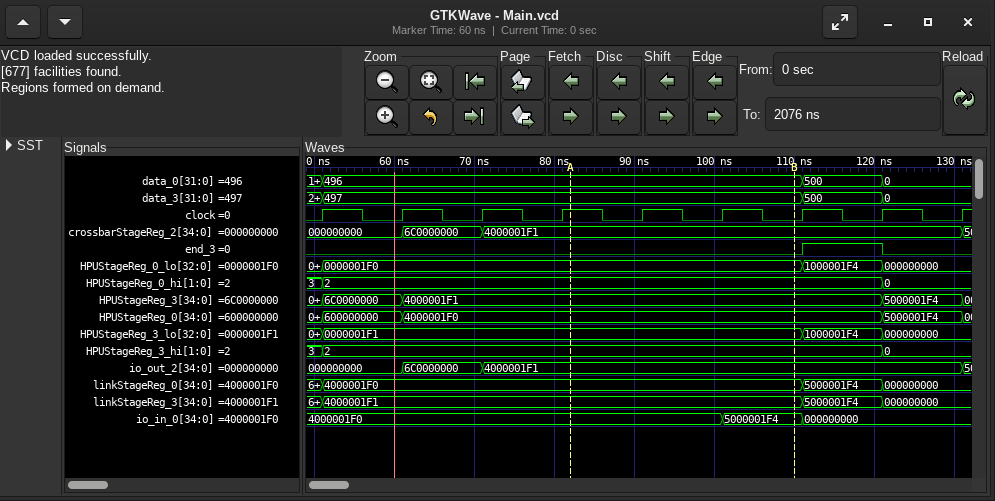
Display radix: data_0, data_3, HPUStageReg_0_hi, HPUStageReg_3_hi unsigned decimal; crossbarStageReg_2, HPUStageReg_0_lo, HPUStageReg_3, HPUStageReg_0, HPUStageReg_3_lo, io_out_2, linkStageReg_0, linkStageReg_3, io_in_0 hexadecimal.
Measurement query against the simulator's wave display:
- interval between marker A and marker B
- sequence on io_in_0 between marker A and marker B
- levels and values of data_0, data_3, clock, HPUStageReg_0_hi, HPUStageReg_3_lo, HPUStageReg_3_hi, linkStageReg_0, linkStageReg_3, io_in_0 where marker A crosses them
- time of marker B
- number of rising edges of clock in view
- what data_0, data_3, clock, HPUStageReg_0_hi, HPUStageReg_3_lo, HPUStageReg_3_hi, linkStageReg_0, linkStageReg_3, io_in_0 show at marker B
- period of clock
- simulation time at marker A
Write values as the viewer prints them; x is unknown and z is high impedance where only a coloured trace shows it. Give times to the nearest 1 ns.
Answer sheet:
28 ns
4000001F0, 5000001F4
data_0=496, data_3=497, clock=1, HPUStageReg_0_hi=2, HPUStageReg_3_lo=0000001F1, HPUStageReg_3_hi=2, linkStageReg_0=4000001F0, linkStageReg_3=4000001F1, io_in_0=4000001F0
110 ns
9
data_0=496, data_3=497, clock=0, HPUStageReg_0_hi=2, HPUStageReg_3_lo=0000001F1, HPUStageReg_3_hi=2, linkStageReg_0=4000001F0, linkStageReg_3=4000001F1, io_in_0=5000001F4
10 ns
82 ns
